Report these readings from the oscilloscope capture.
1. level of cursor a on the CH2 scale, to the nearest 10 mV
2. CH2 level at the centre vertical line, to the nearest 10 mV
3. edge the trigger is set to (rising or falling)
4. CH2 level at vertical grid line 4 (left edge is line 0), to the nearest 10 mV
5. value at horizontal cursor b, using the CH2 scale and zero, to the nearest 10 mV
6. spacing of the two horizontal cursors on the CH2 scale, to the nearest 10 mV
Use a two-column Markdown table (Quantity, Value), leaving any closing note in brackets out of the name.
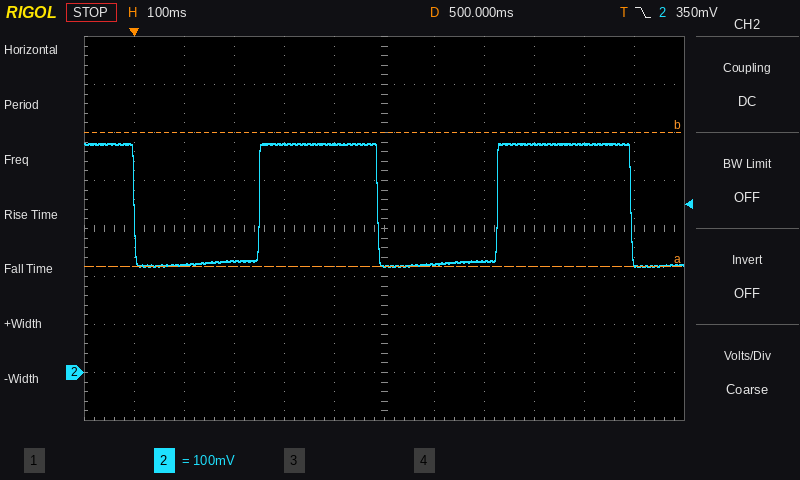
| Quantity | Value |
|---|---|
| level of cursor a on the CH2 scale, to the nearest 10 mV | 220 mV |
| CH2 level at the centre vertical line, to the nearest 10 mV | 220 mV |
| edge the trigger is set to | falling |
| CH2 level at vertical grid line 4 (left edge is line 0), to the nearest 10 mV | 480 mV |
| value at horizontal cursor b, using the CH2 scale and zero, to the nearest 10 mV | 500 mV |
| spacing of the two horizontal cursors on the CH2 scale, to the nearest 10 mV | 280 mV |
